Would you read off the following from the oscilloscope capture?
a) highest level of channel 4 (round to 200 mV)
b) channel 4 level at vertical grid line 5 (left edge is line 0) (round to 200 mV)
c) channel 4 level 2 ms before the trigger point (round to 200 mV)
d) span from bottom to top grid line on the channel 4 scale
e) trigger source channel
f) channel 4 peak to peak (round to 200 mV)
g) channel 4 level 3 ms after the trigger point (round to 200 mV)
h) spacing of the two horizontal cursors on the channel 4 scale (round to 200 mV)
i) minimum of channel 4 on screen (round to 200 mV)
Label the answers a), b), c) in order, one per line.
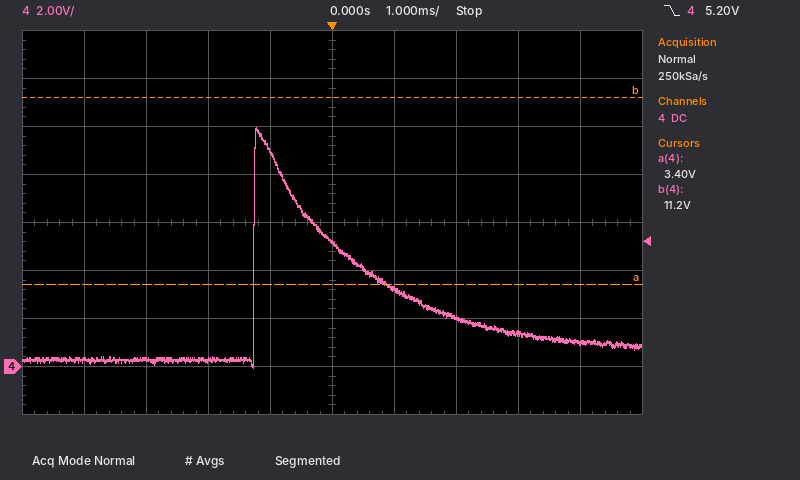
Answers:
a) 10.0 V
b) 5.2 V
c) 200 mV
d) 16 V
e) channel 4
f) 10.0 V
g) 1.4 V
h) 7.8 V
i) 0.0 V
